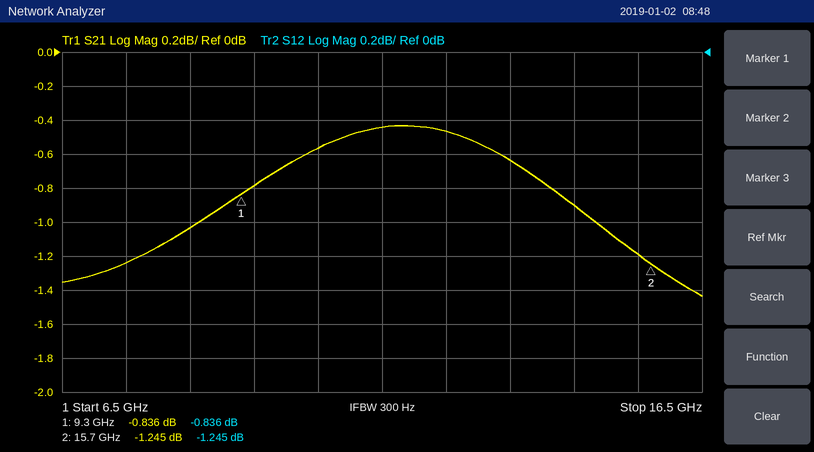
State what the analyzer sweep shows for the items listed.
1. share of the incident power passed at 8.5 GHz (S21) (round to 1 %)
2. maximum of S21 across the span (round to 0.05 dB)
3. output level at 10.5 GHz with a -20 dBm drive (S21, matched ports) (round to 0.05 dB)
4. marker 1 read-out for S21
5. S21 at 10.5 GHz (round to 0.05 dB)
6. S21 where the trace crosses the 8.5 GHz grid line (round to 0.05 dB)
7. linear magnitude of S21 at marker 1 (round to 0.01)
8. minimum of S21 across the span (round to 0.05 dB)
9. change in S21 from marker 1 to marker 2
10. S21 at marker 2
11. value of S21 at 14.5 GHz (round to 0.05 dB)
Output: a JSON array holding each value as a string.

["79 %", "-0.45 dB", "-20.55 dBm", "-0.836 dB", "-0.55 dB", "-1.05 dB", "0.91", "-1.45 dB", "-0.409 dB", "-1.245 dB", "-0.90 dB"]
